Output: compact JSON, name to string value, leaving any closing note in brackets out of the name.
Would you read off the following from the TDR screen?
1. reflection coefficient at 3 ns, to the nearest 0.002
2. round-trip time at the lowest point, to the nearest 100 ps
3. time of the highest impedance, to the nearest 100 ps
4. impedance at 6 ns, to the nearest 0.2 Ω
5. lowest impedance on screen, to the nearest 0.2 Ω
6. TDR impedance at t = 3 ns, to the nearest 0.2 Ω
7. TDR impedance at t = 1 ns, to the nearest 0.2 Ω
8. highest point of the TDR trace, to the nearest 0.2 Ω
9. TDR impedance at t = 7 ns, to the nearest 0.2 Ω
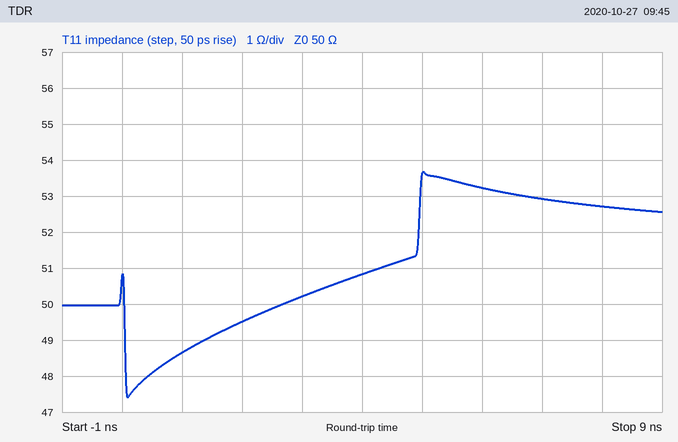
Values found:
{"reflection coefficient at 3 ns, to the nearest 0.002": "+0.002", "round-trip time at the lowest point, to the nearest 100 ps": "100 ps", "time of the highest impedance, to the nearest 100 ps": "5.0 ns", "impedance at 6 ns, to the nearest 0.2 Ω": "53.2 Ω", "lowest impedance on screen, to the nearest 0.2 Ω": "47.4 Ω", "TDR impedance at t = 3 ns, to the nearest 0.2 Ω": "50.2 Ω", "TDR impedance at t = 1 ns, to the nearest 0.2 Ω": "48.6 Ω", "highest point of the TDR trace, to the nearest 0.2 Ω": "53.6 Ω", "TDR impedance at t = 7 ns, to the nearest 0.2 Ω": "53.0 Ω"}
